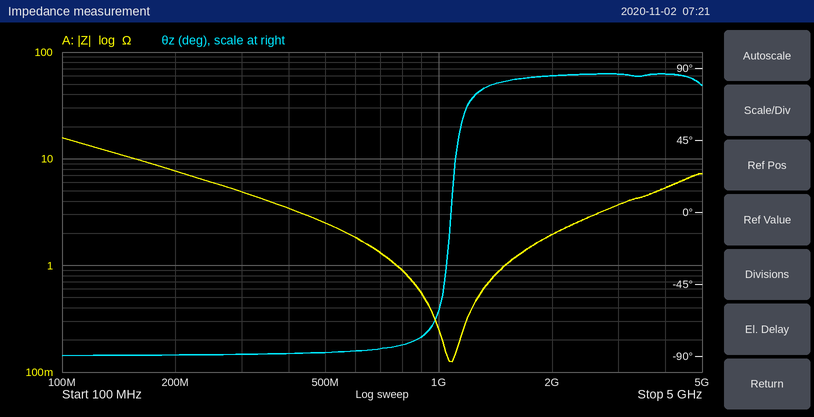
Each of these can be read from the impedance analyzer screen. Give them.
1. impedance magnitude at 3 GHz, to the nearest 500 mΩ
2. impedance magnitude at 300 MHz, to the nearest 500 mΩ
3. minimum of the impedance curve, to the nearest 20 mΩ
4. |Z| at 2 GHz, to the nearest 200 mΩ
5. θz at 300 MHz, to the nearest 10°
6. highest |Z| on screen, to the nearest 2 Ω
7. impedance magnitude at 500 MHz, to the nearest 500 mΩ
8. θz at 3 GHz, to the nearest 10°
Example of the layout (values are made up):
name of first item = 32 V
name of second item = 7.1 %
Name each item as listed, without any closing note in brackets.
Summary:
impedance magnitude at 3 GHz, to the nearest 500 mΩ = 3.5 Ω
impedance magnitude at 300 MHz, to the nearest 500 mΩ = 5.0 Ω
minimum of the impedance curve, to the nearest 20 mΩ = 120 mΩ
|Z| at 2 GHz, to the nearest 200 mΩ = 2.0 Ω
θz at 300 MHz, to the nearest 10° = -90°
highest |Z| on screen, to the nearest 2 Ω = 16 Ω
impedance magnitude at 500 MHz, to the nearest 500 mΩ = 2.5 Ω
θz at 3 GHz, to the nearest 10° = 90°
